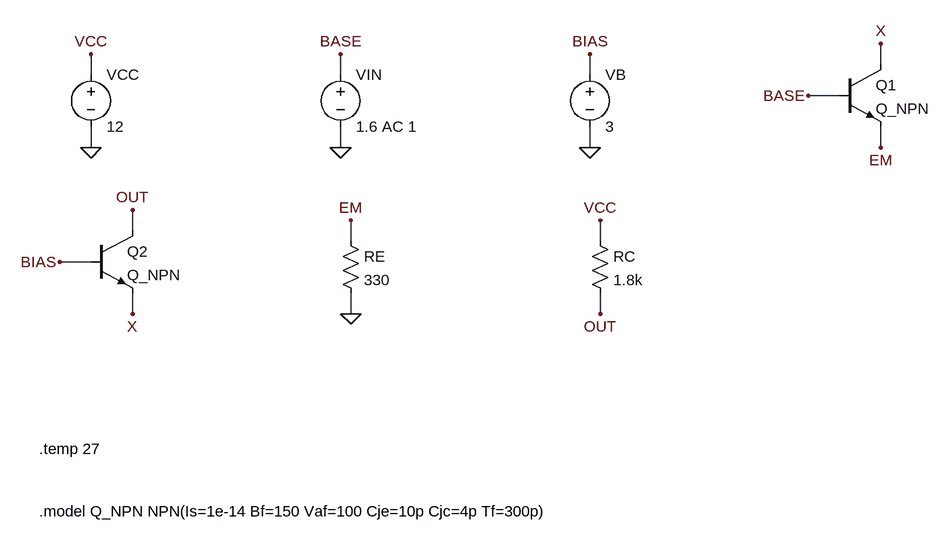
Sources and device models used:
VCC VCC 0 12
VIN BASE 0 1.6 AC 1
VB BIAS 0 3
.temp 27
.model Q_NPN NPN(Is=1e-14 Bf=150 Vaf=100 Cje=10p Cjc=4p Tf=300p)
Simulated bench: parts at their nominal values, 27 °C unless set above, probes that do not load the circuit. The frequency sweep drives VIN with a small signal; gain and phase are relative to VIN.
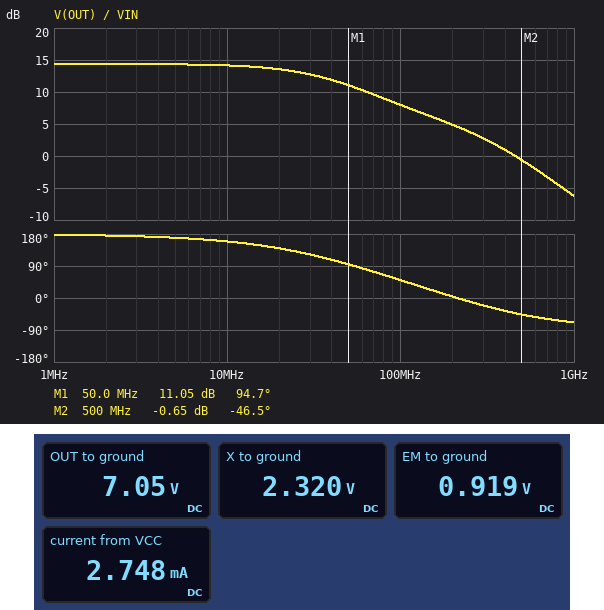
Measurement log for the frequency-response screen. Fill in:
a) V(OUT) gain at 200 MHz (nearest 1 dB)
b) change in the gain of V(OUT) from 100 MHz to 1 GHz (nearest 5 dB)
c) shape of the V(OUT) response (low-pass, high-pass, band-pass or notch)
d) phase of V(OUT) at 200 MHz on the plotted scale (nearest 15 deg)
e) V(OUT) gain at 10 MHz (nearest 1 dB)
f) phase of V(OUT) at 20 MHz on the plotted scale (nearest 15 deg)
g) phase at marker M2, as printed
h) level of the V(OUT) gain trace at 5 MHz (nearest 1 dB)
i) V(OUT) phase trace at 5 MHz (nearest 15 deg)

5 dB
-15 dB
low-pass
0 deg
14 dB
135 deg
-46.5 deg
14 dB
165 deg
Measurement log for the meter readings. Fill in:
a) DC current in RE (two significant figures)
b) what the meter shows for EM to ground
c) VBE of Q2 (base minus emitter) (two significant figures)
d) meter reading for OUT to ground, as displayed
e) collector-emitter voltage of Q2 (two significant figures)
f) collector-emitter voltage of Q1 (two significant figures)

2.8 mA
0.919 V
680 mV
7.05 V
4.7 V
1.4 V
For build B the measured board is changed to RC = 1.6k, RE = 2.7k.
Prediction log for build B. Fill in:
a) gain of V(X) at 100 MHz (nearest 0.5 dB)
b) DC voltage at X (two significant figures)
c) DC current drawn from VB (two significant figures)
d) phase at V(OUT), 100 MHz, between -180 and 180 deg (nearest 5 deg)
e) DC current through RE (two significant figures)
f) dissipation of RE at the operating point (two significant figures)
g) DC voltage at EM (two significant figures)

-19.0 dB
2.4 V
2.2 µA
-10 deg
360 µA
350 µW
970 mV
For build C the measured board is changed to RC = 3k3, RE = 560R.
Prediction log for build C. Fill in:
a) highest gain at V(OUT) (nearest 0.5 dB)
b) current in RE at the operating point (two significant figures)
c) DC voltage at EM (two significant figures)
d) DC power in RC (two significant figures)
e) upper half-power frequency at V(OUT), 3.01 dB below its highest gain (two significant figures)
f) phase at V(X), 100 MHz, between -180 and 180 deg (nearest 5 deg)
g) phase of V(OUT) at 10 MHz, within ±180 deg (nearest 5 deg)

15.0 dB
1.7 mA
930 mV
8.9 mW
24 MHz
100 deg
145 deg
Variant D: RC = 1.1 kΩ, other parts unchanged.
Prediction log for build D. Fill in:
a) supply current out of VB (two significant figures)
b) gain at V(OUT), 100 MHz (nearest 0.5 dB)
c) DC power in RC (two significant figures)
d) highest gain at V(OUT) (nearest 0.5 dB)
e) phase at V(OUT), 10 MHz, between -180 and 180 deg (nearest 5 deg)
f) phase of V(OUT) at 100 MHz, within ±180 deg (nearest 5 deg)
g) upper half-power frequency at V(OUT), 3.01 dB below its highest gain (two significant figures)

17 µA
7.5 dB
8.3 mW
10.0 dB
165 deg
65 deg
120 MHz
